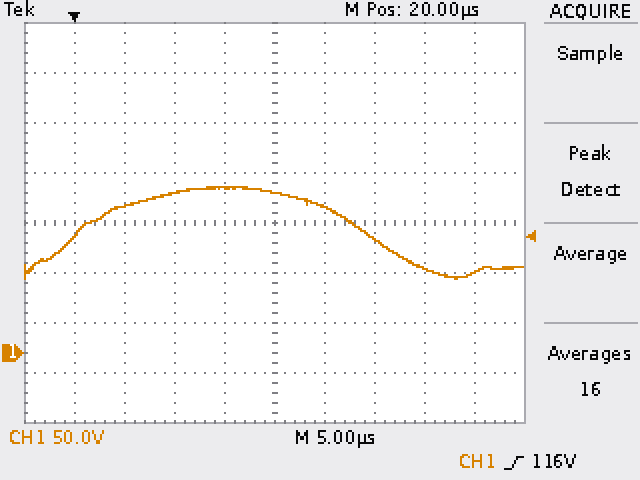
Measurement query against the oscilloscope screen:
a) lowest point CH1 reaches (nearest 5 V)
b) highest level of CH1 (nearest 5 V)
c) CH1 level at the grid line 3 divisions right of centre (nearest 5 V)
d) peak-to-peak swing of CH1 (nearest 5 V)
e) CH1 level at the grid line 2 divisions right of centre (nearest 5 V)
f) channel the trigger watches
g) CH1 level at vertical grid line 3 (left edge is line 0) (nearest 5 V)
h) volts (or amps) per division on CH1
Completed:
75 V
165 V
85 V
90 V
115 V
CH1
160 V
50 V
